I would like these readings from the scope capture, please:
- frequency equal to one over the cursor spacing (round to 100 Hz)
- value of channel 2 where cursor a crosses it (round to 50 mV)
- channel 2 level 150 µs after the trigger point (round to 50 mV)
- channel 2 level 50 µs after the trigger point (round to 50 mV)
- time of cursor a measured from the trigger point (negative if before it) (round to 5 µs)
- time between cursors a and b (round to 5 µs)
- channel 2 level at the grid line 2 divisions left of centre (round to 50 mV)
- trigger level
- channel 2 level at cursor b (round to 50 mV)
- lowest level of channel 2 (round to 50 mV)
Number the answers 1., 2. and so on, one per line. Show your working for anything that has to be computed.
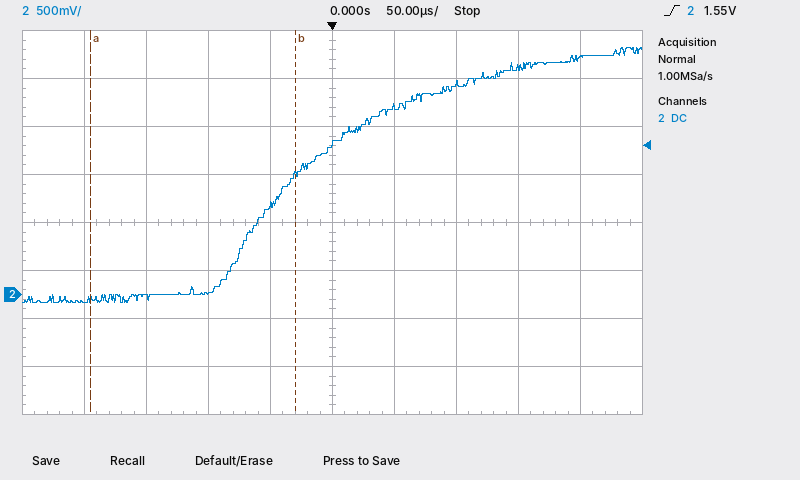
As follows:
1. 1 / 165 µs ≈ 6.1 kHz
2. -50 mV
3. 2.35 V
4. 1.95 V
5. -195 µs
6. 165 µs
7. 0 mV
8. 1.55 V
9. 1.25 V
10. -100 mV
